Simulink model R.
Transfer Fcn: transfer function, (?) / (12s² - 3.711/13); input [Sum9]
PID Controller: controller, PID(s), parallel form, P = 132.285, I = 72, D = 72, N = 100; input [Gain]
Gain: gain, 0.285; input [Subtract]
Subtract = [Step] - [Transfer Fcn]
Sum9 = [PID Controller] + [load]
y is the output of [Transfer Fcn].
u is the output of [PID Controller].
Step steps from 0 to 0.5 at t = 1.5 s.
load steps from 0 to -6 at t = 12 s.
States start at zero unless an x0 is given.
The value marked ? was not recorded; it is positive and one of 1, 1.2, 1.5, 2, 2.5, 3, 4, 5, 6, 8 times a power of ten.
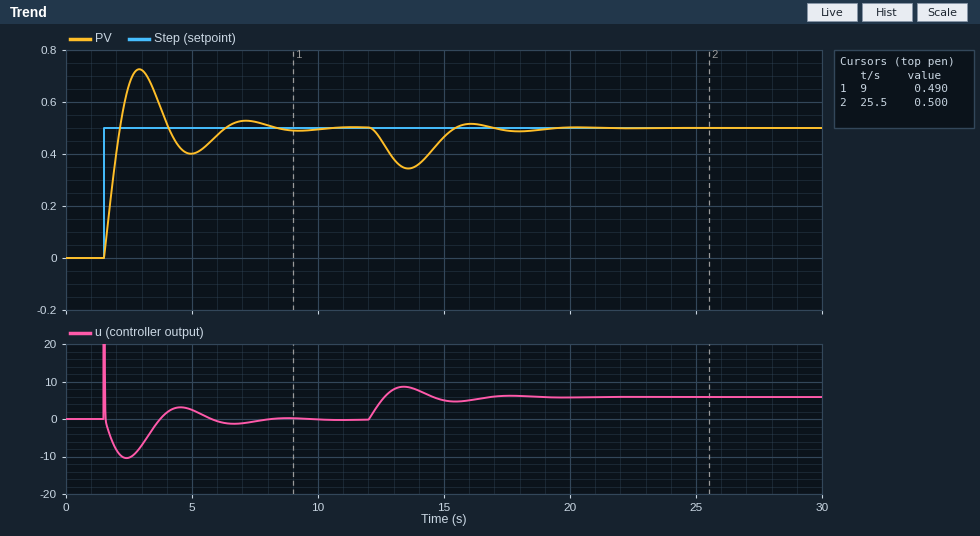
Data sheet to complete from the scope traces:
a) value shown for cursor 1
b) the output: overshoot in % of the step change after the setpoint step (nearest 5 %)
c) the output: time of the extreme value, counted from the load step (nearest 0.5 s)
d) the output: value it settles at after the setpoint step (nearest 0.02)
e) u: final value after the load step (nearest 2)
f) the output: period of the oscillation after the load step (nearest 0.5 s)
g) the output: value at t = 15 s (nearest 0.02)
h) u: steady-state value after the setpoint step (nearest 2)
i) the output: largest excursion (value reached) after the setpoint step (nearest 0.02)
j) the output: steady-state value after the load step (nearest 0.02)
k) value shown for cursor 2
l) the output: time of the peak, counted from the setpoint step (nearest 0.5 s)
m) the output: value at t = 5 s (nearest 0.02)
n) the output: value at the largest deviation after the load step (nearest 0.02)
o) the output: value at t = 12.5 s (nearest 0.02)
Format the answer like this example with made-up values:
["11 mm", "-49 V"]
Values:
["0.490", "45 %", "1.5 s", "0.50", "6", "4.5 s", "0.46", "0", "0.72", "0.50", "0.500", "1.5 s", "0.40", "0.34", "0.46"]
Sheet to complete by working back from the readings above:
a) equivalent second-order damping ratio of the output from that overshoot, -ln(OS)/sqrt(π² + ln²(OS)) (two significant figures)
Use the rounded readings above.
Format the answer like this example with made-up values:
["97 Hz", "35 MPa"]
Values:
["0.25"]
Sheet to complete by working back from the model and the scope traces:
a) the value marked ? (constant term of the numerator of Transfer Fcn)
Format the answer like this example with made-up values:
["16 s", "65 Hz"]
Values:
["1"]
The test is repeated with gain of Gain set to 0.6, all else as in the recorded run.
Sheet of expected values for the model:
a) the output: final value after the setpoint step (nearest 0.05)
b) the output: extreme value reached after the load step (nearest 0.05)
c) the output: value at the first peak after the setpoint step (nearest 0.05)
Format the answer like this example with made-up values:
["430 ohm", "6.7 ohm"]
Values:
["0.50", "0.45", "0.65"]
